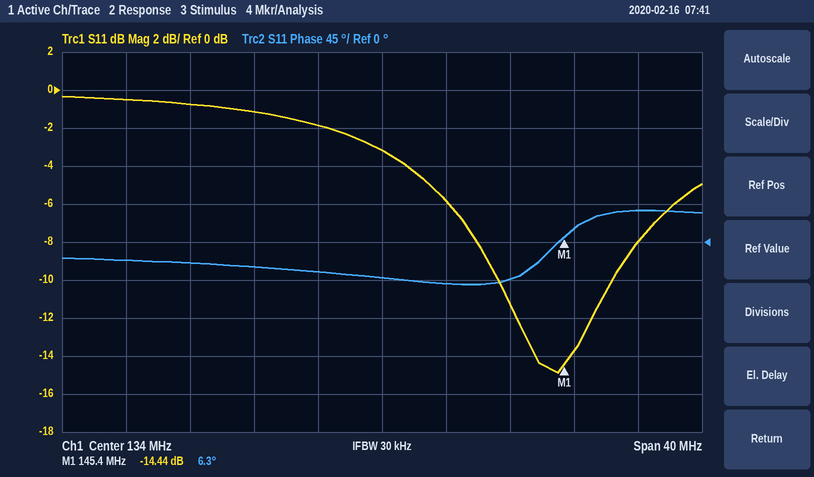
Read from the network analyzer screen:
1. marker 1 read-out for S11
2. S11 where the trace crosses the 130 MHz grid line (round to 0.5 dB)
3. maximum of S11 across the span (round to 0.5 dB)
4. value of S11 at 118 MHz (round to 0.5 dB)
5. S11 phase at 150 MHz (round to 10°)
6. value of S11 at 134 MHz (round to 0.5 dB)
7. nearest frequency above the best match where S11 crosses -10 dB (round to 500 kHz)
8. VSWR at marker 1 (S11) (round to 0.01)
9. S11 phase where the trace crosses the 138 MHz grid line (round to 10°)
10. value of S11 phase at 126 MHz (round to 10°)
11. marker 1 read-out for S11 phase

-14.44 dB
-2.0 dB
-0.5 dB
-0.5 dB
40°
-3.0 dB
148.5 MHz
1.47
-50°
-30°
6.3°
